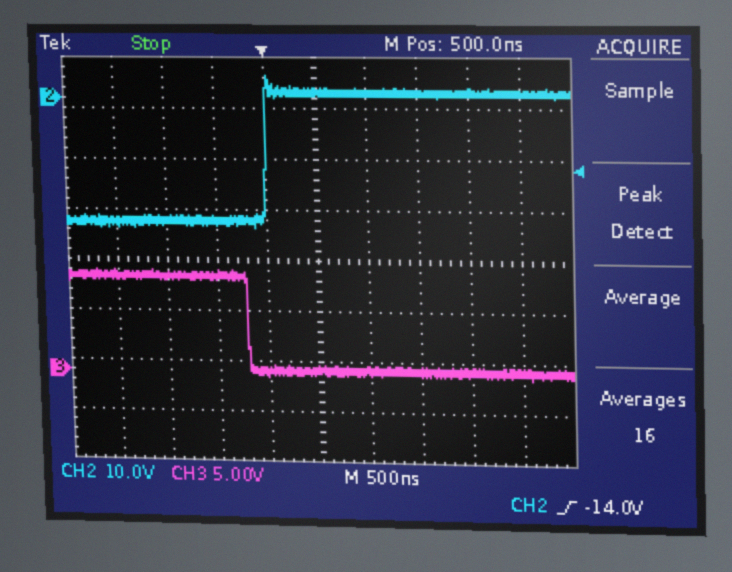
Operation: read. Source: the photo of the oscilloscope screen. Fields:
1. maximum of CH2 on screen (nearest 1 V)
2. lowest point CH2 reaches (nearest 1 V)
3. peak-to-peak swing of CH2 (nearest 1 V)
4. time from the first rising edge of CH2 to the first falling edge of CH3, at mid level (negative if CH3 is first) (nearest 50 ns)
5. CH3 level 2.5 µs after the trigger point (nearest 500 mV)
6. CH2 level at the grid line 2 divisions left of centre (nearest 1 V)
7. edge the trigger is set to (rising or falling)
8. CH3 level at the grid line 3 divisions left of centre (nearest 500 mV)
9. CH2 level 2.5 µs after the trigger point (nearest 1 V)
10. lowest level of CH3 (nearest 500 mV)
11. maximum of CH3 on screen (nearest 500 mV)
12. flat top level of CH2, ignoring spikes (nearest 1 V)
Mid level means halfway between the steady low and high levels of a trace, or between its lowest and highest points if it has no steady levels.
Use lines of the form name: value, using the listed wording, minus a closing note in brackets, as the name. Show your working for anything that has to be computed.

maximum of CH2 on screen: 4 V
lowest point CH2 reaches: -26 V
peak-to-peak swing of CH2: 4 V − (-26 V) = 30 V
time from the first rising edge of CH2 to the first falling edge of CH3, at mid level (negative if CH3 is first): -200 ns
CH3 level 2.5 µs after the trigger point: 0.0 V
CH2 level at the grid line 2 divisions left of centre: -24 V
edge the trigger is set to: rising
CH3 level at the grid line 3 divisions left of centre: 9.5 V
CH2 level 2.5 µs after the trigger point: 1 V
lowest level of CH3: -500 mV
maximum of CH3 on screen: 10.0 V
flat top level of CH2, ignoring spikes: 1 V
